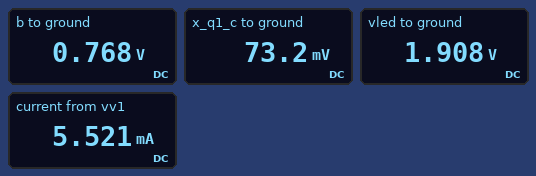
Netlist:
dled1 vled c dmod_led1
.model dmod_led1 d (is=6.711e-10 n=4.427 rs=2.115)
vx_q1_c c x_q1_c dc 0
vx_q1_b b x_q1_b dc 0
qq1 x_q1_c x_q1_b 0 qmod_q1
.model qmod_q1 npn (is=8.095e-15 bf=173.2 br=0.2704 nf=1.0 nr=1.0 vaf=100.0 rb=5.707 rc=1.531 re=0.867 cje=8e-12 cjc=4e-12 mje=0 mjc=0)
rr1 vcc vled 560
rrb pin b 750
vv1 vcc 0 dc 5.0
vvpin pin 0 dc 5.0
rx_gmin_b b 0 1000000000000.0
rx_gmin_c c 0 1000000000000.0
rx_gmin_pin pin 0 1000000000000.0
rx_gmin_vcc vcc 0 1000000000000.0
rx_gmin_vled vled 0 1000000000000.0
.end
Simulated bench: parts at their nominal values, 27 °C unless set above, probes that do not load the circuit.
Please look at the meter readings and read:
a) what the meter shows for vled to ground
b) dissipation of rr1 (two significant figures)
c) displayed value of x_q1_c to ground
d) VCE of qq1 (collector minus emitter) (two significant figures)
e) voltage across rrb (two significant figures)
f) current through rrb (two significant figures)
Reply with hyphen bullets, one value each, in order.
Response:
- 1.908 V
- 17 mW
- 73.2 mV
- 73 mV
- 4.2 V
- 5.6 mA
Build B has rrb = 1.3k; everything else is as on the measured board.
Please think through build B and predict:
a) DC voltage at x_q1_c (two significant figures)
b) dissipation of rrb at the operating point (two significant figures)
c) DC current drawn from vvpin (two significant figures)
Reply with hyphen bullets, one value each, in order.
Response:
- 78 mV
- 14 mW
- 3.3 mA
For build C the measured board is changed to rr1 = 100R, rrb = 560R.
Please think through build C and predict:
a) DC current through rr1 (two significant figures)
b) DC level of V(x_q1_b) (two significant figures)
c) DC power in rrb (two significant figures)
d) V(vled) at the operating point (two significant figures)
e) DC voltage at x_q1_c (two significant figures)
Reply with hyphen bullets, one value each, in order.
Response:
- 28 mA
- 830 mV
- 31 mW
- 2.2 V
- 150 mV
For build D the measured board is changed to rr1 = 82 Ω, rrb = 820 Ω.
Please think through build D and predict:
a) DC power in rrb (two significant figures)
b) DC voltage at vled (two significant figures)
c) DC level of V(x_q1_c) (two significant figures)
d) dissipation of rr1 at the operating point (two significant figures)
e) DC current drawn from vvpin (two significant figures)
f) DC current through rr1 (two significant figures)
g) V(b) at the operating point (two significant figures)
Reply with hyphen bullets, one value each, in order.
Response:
- 21 mW
- 2.3 V
- 170 mV
- 91 mW
- 5.1 mA
- 33 mA
- 820 mV
